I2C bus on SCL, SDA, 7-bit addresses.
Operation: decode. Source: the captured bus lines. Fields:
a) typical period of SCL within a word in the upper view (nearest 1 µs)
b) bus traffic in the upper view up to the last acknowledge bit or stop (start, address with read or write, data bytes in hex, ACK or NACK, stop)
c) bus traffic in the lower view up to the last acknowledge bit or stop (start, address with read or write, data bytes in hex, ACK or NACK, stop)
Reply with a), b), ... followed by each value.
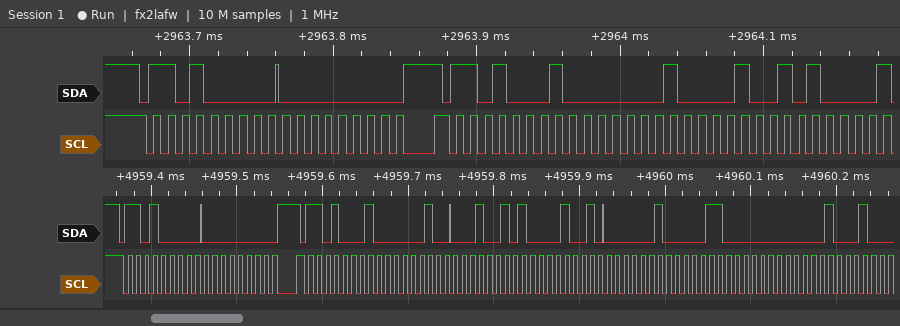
a) 10 µs
b) start, address 68 write ACK, 00 ACK, repeated start, address 68 read ACK, 02 ACK, 25 ACK
c) start, address 68 write ACK, 00 ACK, repeated start, address 68 read ACK, 04 ACK, 25 ACK, 12 ACK, 04 ACK, 30 ACK, 01 ACK
